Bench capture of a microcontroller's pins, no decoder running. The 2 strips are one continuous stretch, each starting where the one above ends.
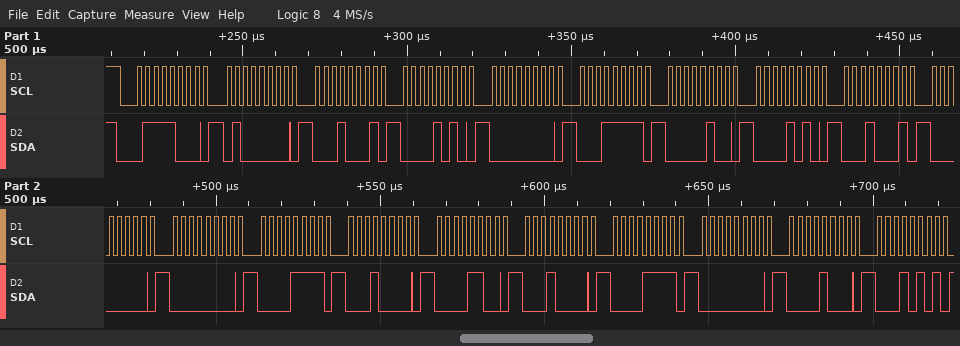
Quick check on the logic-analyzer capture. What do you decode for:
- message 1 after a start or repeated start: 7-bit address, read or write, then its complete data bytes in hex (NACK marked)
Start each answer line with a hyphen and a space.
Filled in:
- 0x3C write: 40 11 0A 00 1F 04 0A 11 00 00 0F 10 0C 10 0F 00 08 15
